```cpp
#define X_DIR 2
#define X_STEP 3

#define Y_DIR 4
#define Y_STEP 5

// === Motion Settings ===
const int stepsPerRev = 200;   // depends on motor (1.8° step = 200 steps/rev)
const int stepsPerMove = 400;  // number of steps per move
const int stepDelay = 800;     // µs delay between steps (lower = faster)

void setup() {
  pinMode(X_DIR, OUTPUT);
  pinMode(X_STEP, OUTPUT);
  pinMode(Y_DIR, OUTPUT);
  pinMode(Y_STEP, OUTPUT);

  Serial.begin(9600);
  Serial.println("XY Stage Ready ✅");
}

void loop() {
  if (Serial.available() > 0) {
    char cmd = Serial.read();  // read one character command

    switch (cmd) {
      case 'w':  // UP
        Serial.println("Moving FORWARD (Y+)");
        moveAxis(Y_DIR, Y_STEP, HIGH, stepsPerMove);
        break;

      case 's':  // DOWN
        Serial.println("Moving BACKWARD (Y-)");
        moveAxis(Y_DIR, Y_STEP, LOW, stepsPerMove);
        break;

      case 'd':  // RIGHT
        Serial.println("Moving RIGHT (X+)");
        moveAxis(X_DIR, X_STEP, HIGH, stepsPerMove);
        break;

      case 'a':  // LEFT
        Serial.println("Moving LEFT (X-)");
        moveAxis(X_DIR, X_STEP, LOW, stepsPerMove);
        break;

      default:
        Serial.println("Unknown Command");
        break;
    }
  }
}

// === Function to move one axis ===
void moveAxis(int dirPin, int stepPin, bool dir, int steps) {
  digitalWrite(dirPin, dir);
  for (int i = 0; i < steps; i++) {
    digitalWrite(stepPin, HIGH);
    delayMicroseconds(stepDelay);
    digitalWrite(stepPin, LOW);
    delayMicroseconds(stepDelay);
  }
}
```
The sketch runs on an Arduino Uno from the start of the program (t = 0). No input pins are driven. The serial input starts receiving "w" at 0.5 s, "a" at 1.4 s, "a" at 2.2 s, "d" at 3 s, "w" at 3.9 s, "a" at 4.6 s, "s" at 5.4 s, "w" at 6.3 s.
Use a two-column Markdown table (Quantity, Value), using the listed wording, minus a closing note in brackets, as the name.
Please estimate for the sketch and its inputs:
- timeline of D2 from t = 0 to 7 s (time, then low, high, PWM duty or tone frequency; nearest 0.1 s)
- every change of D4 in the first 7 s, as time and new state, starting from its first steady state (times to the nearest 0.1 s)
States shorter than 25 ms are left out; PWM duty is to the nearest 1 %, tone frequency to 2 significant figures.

| Quantity | Value |
|---|---|
| timeline of D2 from t = 0 to 7 s | 0 s low; 3 s high; 4.6 s low |
| every change of D4 in the first 7 s, as time and new state, starting from its first steady state | 0 s low; 0.5 s high; 5.4 s low; 6.3 s high |
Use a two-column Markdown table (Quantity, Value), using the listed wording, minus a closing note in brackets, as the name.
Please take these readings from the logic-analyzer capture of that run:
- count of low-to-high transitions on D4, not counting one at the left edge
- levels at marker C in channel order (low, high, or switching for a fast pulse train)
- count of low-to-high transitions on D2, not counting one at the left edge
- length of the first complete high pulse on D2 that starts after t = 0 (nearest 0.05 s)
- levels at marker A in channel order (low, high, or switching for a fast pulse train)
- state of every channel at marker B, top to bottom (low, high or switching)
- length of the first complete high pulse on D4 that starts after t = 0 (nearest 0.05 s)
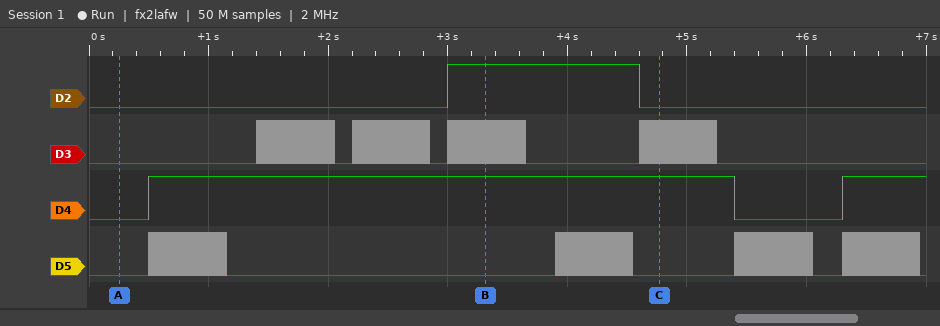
| Quantity | Value |
|---|---|
| count of low-to-high transitions on D4, not counting one at the left edge | 2 |
| levels at marker C in channel order | D2 low, D3 switching, D4 high, D5 low |
| count of low-to-high transitions on D2, not counting one at the left edge | 1 |
| length of the first complete high pulse on D2 that starts after t = 0 | 1.60 s |
| levels at marker A in channel order | D2 low, D3 low, D4 low, D5 low |
| state of every channel at marker B, top to bottom | D2 high, D3 switching, D4 high, D5 low |
| length of the first complete high pulse on D4 that starts after t = 0 | 4.90 s |
